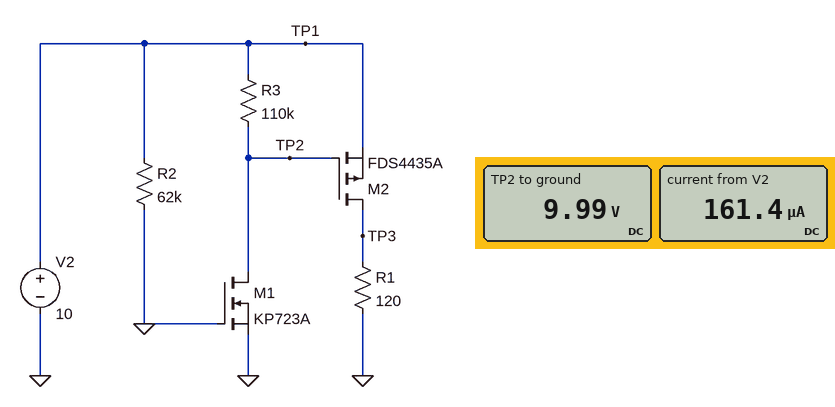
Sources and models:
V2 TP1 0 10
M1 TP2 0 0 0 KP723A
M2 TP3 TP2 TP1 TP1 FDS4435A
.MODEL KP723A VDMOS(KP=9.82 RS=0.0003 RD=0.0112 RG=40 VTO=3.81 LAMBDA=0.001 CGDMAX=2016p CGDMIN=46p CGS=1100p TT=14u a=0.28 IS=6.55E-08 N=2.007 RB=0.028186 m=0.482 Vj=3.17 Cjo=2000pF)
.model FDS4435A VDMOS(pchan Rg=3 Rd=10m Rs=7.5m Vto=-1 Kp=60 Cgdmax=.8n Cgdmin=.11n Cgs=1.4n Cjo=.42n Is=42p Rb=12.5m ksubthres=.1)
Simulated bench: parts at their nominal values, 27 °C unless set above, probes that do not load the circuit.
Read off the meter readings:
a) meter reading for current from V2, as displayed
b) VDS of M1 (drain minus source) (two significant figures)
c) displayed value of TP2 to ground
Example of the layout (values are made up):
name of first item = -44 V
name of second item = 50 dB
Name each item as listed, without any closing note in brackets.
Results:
meter reading for current from V2, as displayed = 161.4 µA
VDS of M1 (drain minus source) = 10 V
displayed value of TP2 to ground = 9.99 V
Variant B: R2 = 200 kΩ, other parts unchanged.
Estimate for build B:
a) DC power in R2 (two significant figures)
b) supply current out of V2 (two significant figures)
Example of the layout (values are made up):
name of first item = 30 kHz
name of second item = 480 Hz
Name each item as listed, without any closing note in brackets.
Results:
DC power in R2 = 500 µW
supply current out of V2 = 50 µA
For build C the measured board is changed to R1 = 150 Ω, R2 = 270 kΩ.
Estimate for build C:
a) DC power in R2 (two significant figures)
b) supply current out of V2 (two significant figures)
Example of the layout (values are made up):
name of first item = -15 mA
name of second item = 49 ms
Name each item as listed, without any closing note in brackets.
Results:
DC power in R2 = 370 µW
supply current out of V2 = 37 µA
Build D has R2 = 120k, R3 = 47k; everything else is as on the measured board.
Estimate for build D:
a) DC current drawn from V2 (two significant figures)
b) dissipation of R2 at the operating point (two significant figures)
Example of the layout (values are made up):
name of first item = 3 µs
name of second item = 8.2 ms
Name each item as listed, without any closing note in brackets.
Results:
DC current drawn from V2 = 83 µA
dissipation of R2 at the operating point = 830 µW
